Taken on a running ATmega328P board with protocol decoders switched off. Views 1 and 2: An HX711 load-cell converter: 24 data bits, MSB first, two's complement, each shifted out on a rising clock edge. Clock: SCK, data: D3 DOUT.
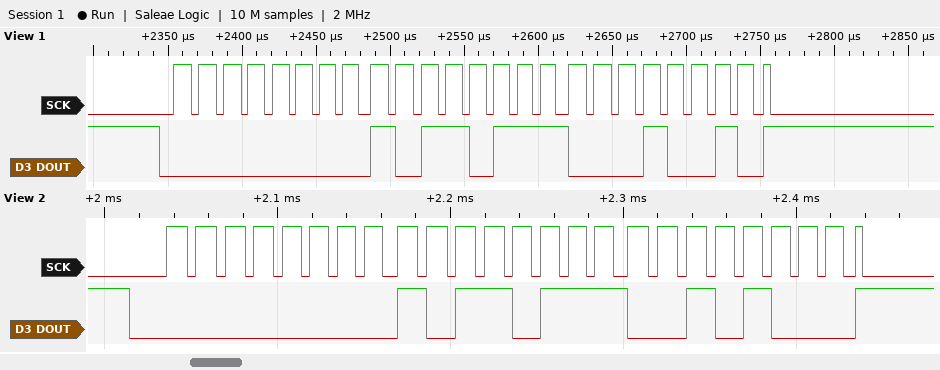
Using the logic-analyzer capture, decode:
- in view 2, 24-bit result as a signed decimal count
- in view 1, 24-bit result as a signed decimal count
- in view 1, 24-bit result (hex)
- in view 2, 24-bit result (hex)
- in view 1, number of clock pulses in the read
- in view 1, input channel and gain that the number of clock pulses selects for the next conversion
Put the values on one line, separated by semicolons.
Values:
46888; 46866; 0x00B712; 0x00B728; 25; channel A, gain 128
